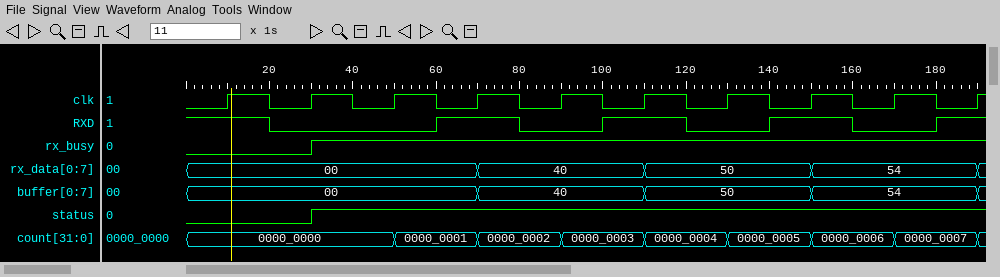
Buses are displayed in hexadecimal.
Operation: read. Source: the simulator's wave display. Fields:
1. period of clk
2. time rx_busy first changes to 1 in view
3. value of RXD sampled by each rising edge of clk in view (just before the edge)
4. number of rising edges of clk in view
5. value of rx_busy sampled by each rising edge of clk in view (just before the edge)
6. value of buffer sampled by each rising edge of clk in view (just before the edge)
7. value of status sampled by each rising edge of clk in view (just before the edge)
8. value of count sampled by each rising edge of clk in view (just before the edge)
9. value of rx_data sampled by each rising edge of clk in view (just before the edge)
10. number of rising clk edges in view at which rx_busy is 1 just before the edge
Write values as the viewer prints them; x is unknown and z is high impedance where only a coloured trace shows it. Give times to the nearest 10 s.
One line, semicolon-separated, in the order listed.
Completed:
20 s; 30 s; 1 0 0 1 0 1 0 1 0 1; 10; 0 0 1 1 1 1 1 1 1 1; 00, 00, 00, 00, 40, 40, 50, 50, 54, 54; 0 0 1 1 1 1 1 1 1 1; 0000_0000, 0000_0000, 0000_0000, 0000_0001, 0000_0002, 0000_0003, 0000_0004, 0000_0005, 0000_0006, 0000_0007; 00, 00, 00, 00, 40, 40, 50, 50, 54, 54; 8
